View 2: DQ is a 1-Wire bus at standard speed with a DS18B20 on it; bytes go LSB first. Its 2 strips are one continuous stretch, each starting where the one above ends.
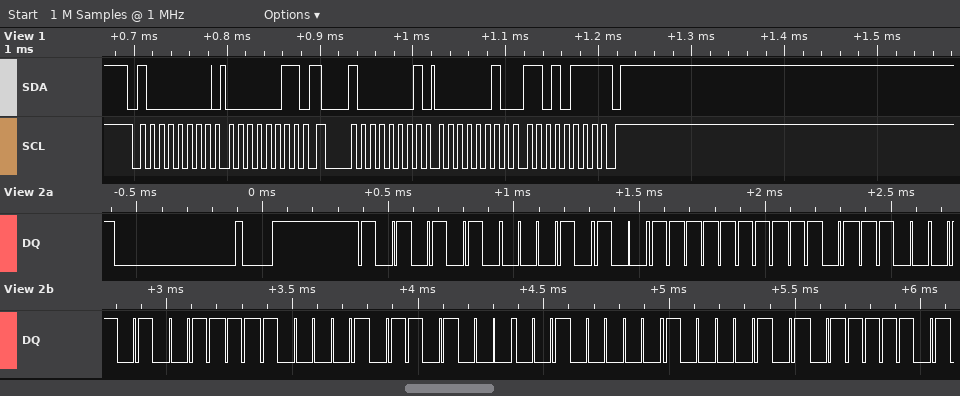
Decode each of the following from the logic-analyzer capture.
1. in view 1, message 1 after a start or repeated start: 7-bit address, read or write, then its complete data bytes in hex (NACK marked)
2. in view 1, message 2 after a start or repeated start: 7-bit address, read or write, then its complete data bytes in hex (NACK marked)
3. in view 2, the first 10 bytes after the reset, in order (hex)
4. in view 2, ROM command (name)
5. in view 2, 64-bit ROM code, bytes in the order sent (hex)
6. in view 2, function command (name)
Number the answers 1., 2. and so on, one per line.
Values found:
1. 0x40 write: 03
2. 0x40 read: 02 D7 NACK
3. 55 28 FF 3B CA 87 16 04 A1 BE
4. Match ROM
5. 28 FF 3B CA 87 16 04 A1
6. Read Scratchpad
